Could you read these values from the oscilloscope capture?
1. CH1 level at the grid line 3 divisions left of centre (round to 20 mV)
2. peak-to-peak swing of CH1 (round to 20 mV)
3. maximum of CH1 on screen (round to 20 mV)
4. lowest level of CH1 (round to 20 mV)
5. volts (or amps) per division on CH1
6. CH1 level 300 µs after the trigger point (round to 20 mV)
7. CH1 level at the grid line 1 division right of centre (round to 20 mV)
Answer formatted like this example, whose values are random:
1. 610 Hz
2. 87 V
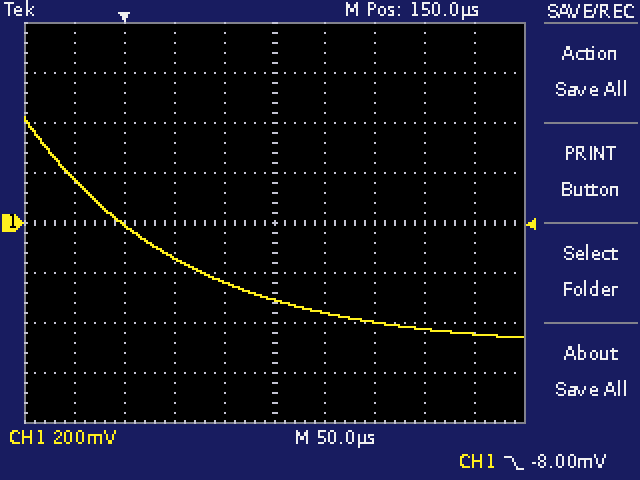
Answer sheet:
1. 0 mV
2. 880 mV
3. 420 mV
4. -460 mV
5. 200 mV
6. -420 mV
7. -360 mV
